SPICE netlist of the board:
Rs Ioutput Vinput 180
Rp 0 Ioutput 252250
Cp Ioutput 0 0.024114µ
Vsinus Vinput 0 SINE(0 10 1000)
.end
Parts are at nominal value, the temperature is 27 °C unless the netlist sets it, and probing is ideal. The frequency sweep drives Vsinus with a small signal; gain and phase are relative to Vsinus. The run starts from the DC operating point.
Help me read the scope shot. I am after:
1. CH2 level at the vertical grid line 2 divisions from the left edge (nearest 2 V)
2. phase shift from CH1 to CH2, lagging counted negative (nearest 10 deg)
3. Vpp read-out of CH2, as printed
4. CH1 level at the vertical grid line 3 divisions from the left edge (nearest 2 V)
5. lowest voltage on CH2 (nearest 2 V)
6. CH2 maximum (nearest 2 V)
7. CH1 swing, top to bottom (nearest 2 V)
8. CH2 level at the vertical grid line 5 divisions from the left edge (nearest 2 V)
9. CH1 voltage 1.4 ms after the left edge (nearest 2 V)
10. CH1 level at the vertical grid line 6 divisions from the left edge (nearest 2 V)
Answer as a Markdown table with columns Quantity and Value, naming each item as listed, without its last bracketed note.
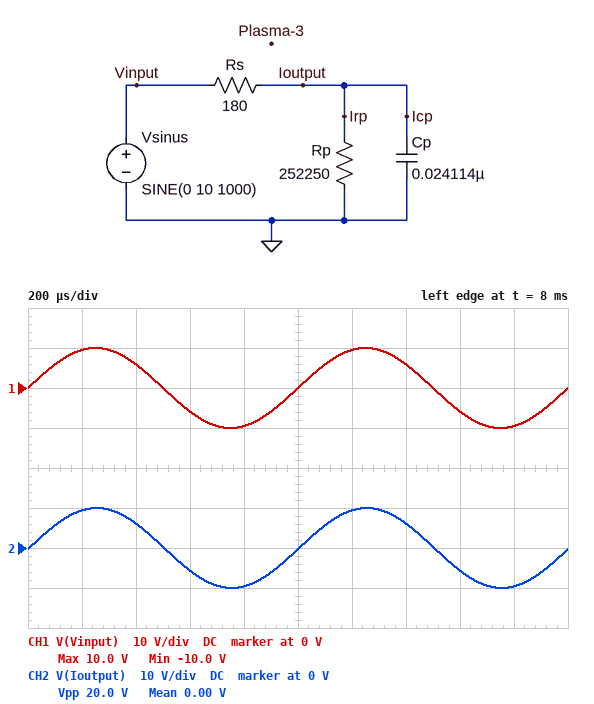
| Quantity | Value |
|---|---|
| CH2 level at the vertical grid line 2 divisions from the left edge | 6 V |
| phase shift from CH1 to CH2, lagging counted negative | 0 deg |
| Vpp read-out of CH2, as printed | 20.0 V |
| CH1 level at the vertical grid line 3 divisions from the left edge | -6 V |
| lowest voltage on CH2 | -10 V |
| CH2 maximum | 10 V |
| CH1 swing, top to bottom | 20 V |
| CH2 level at the vertical grid line 5 divisions from the left edge | 0 V |
| CH1 voltage 1.4 ms after the left edge | 6 V |
| CH1 level at the vertical grid line 6 divisions from the left edge | 10 V |
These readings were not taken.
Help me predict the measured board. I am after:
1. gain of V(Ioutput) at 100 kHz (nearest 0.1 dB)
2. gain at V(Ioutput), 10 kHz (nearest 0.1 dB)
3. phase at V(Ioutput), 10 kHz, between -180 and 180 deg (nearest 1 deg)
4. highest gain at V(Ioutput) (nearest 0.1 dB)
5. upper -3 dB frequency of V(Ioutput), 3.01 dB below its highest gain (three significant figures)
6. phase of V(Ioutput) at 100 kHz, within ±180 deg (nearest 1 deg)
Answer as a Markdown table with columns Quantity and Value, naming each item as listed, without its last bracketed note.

| Quantity | Value |
|---|---|
| gain of V(Ioutput) at 100 kHz | -9.3 dB |
| gain at V(Ioutput), 10 kHz | -0.3 dB |
| phase at V(Ioutput), 10 kHz, between -180 and 180 deg | -15 deg |
| highest gain at V(Ioutput) | 0 dB |
| upper -3 dB frequency of V(Ioutput), 3.01 dB below its highest gain | 36.7 kHz |
| phase of V(Ioutput) at 100 kHz, within ±180 deg | -70 deg |
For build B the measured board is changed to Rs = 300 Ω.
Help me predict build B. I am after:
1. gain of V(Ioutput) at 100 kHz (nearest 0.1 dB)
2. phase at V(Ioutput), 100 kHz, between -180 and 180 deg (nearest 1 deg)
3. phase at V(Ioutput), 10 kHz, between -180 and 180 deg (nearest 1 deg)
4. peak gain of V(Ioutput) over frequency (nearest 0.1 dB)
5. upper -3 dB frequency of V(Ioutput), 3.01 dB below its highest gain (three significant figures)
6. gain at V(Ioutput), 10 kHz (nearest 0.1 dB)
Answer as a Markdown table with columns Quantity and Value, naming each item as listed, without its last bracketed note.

| Quantity | Value |
|---|---|
| gain of V(Ioutput) at 100 kHz | -13.4 dB |
| phase at V(Ioutput), 100 kHz, between -180 and 180 deg | -78 deg |
| phase at V(Ioutput), 10 kHz, between -180 and 180 deg | -24 deg |
| peak gain of V(Ioutput) over frequency | 0 dB |
| upper -3 dB frequency of V(Ioutput), 3.01 dB below its highest gain | 22.0 kHz |
| gain at V(Ioutput), 10 kHz | -0.8 dB |
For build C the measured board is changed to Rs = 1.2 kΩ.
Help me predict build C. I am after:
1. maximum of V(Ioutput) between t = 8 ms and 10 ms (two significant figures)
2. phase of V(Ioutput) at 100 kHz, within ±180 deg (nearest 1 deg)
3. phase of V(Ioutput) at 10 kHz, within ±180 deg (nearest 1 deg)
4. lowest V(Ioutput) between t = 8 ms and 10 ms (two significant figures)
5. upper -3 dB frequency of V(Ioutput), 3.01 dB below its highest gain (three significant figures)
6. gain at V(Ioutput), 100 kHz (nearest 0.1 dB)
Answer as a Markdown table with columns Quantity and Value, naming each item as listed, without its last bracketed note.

| Quantity | Value |
|---|---|
| maximum of V(Ioutput) between t = 8 ms and 10 ms | 9.8 V |
| phase of V(Ioutput) at 100 kHz, within ±180 deg | -87 deg |
| phase of V(Ioutput) at 10 kHz, within ±180 deg | -61 deg |
| lowest V(Ioutput) between t = 8 ms and 10 ms | -9.8 V |
| upper -3 dB frequency of V(Ioutput), 3.01 dB below its highest gain | 5.53 kHz |
| gain at V(Ioutput), 100 kHz | -25.2 dB |
